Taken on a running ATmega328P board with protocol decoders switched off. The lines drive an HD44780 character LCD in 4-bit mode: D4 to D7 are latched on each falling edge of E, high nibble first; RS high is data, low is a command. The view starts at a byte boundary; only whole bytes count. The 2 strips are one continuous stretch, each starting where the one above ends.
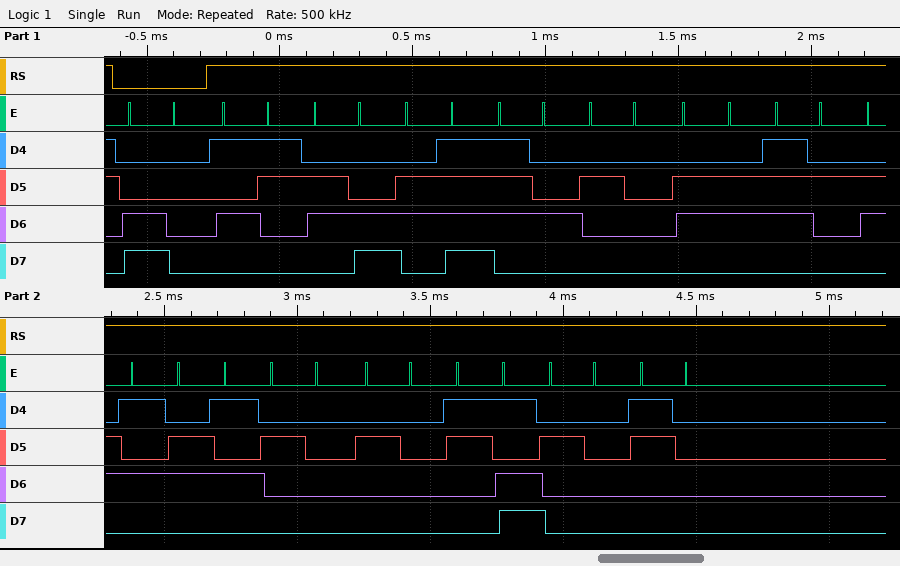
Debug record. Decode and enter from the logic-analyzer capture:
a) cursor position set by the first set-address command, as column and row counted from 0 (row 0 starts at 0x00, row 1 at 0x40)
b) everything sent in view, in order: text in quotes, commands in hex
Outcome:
column 0, row 1
0xC0 "Slot free  = 0"
